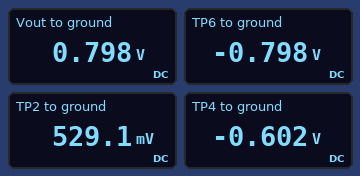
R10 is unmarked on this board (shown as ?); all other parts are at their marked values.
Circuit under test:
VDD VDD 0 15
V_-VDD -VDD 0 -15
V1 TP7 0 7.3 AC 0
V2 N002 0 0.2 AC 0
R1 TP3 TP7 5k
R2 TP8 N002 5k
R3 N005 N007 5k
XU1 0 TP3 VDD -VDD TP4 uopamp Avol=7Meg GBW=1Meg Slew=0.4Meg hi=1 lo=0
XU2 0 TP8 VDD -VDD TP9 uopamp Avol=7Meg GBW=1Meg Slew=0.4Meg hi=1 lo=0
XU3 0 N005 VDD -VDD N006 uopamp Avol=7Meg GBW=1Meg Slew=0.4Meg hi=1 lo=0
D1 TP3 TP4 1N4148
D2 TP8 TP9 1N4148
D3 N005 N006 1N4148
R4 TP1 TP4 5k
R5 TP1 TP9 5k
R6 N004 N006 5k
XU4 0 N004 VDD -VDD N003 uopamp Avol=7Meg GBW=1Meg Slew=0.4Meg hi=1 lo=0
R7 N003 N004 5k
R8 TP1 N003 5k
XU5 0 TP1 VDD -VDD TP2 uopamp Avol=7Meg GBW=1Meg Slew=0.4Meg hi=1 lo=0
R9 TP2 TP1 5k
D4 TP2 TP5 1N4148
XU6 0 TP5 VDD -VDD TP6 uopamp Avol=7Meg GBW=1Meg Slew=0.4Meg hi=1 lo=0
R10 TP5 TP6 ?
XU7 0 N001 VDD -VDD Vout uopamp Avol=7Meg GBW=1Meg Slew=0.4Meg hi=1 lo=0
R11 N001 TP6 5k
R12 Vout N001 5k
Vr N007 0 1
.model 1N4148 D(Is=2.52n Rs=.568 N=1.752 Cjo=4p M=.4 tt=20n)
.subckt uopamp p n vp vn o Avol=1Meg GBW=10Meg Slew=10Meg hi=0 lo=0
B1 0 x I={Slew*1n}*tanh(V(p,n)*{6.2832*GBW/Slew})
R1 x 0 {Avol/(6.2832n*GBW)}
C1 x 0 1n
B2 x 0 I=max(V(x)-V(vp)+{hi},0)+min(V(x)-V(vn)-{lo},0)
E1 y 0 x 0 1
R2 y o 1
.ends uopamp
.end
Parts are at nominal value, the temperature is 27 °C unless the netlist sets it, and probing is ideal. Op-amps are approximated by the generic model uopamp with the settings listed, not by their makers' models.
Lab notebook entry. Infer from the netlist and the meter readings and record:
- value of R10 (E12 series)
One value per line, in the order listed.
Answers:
2.7 kΩ
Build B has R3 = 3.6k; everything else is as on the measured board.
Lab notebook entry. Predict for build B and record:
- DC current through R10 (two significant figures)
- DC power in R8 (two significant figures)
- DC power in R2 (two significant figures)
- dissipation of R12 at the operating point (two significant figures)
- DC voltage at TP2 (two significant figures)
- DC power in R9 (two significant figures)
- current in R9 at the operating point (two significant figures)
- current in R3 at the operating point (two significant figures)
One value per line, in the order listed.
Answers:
210 µA
55 µW
8.0 µW
66 µW
510 mV
53 µW
100 µA
280 µA
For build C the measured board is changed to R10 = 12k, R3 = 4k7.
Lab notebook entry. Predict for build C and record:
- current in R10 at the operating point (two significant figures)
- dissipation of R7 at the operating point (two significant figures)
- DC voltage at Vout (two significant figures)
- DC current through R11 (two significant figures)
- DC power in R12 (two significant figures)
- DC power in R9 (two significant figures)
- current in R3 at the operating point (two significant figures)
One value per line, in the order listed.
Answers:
280 µA
53 µW
3.3 V
670 µA
2.2 mW
55 µW
210 µA
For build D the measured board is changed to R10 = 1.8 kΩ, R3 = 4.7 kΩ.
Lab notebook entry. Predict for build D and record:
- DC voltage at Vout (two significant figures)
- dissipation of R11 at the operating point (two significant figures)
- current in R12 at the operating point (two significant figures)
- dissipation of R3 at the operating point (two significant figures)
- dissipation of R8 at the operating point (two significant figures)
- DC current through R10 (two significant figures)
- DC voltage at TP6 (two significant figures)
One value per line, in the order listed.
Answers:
500 mV
50 µW
100 µA
210 µW
53 µW
280 µA
-500 mV
